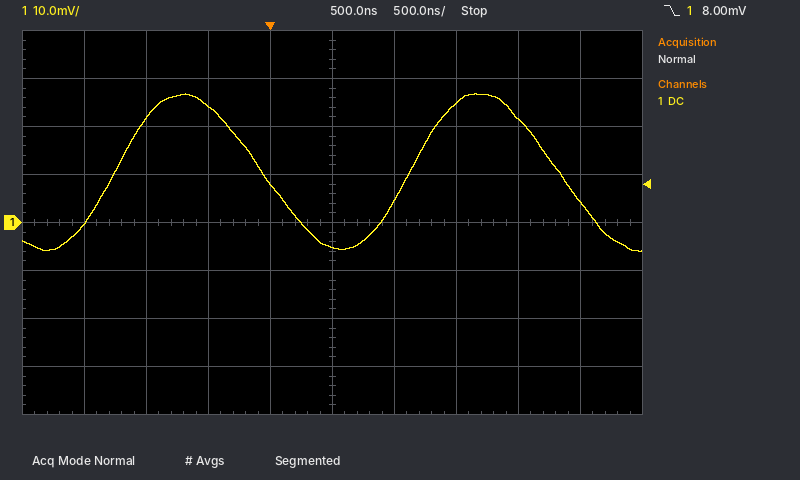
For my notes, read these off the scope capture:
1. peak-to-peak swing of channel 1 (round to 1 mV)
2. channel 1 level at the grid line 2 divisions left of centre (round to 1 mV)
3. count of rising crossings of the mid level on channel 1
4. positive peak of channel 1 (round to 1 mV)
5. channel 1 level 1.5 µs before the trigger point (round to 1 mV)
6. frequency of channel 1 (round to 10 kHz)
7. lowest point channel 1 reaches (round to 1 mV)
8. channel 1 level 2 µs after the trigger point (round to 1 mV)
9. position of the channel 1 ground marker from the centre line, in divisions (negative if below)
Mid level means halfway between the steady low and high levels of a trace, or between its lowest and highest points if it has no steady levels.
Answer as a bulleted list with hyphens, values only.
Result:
- 33 mV
- 24 mV
- 2
- 27 mV
- 0 mV
- 420 kHz
- -6 mV
- 22 mV
- 0.0 div
